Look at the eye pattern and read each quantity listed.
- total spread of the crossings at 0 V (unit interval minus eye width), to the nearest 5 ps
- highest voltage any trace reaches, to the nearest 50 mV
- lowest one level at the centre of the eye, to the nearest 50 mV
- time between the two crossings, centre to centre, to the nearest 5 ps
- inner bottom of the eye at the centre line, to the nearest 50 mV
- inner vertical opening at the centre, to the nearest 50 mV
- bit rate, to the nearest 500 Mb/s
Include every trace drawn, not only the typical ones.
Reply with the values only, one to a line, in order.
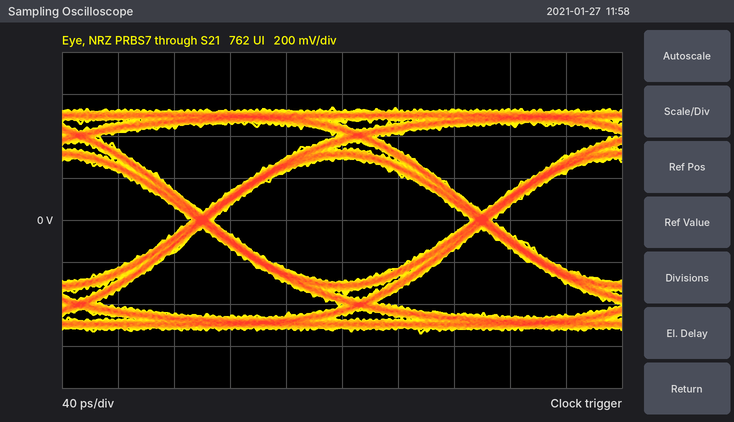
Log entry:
15 ps
550 mV
300 mV
200 ps
-300 mV
600 mV
5.0 Gb/s
